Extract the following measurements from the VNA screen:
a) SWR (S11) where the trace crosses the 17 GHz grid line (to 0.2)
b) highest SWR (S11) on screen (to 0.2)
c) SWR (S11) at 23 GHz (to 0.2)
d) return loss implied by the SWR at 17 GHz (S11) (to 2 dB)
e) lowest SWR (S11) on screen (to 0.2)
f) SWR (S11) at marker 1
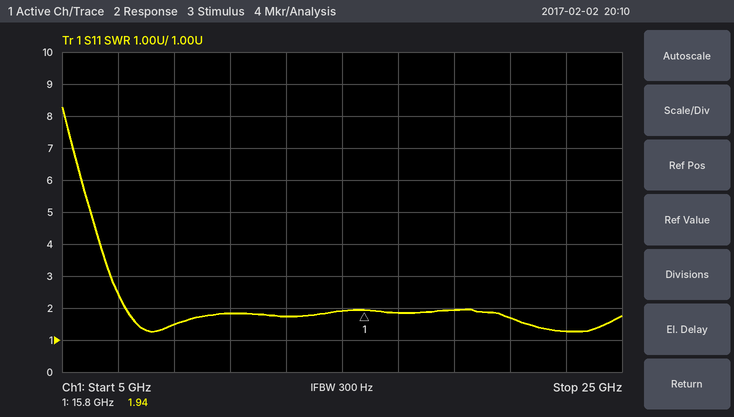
1.8
8.2
1.2
10 dB
1.2
1.94
